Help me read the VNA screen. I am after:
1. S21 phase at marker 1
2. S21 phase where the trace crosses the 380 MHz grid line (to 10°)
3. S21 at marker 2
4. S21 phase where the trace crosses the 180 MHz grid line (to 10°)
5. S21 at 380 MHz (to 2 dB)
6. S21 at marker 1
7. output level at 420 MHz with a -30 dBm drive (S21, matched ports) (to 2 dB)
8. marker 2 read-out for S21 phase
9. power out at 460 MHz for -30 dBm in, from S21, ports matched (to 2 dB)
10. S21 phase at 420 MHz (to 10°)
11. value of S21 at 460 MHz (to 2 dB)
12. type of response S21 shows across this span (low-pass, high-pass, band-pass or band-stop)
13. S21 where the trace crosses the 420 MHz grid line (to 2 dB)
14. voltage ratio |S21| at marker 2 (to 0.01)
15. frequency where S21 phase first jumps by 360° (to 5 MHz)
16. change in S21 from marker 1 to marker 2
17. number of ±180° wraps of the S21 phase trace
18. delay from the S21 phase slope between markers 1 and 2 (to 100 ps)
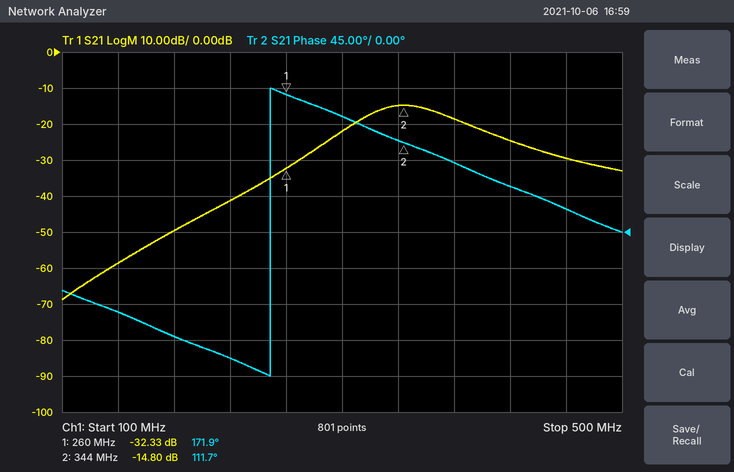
171.9°
90°
-14.80 dB
-130°
-18 dB
-32.33 dB
-54 dBm
111.7°
-60 dBm
60°
-30 dB
band-pass
-24 dB
0.18
250 MHz
17.53 dB
1
2.0 ns
